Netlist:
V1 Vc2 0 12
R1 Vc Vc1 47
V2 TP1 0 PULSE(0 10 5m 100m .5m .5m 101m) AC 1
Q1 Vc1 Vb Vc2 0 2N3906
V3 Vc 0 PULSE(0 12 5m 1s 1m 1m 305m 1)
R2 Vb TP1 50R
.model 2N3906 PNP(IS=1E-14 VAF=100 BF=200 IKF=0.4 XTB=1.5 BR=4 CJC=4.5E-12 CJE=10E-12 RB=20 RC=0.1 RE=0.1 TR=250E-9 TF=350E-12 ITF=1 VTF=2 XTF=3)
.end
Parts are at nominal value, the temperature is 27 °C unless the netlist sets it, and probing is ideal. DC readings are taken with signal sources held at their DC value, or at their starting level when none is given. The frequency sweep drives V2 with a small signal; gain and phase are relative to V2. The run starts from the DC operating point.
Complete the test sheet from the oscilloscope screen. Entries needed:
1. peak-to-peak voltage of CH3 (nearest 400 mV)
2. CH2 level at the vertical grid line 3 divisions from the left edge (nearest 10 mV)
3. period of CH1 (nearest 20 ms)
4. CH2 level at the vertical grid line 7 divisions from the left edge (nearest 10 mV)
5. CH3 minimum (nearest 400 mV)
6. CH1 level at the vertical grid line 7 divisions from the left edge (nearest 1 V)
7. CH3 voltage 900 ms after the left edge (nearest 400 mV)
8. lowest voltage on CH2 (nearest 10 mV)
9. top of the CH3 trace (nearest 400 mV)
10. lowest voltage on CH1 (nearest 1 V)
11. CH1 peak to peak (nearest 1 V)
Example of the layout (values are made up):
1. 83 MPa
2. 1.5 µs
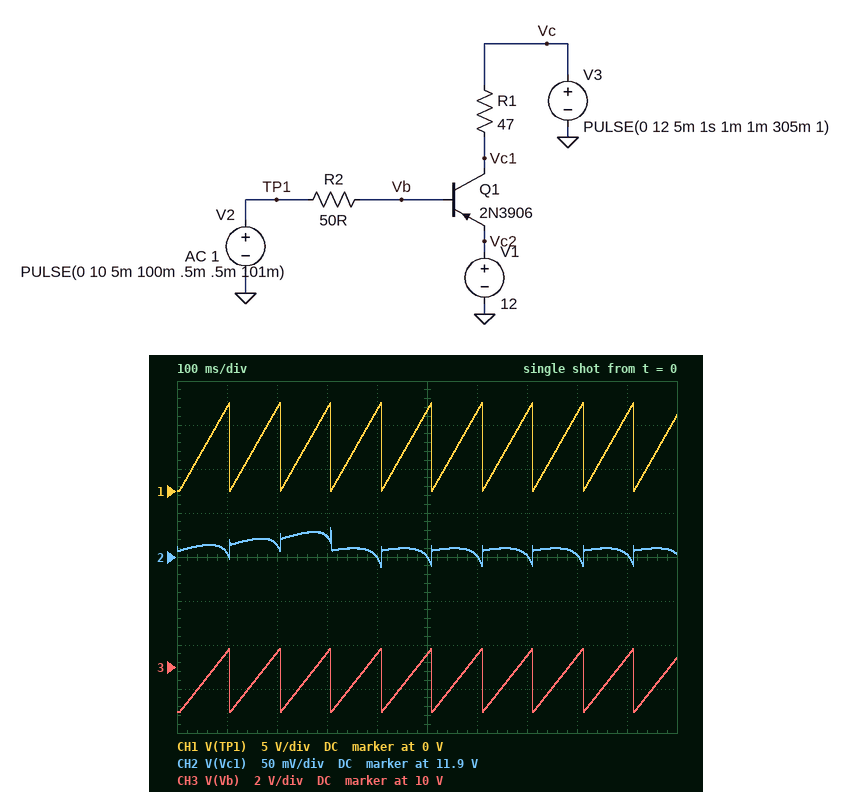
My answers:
1. 2.8 V
2. 11.92 V
3. 100 ms
4. 11.90 V
5. 8.0 V
6. 9 V
7. 10.4 V
8. 11.89 V
9. 10.8 V
10. 0 V
11. 10 V
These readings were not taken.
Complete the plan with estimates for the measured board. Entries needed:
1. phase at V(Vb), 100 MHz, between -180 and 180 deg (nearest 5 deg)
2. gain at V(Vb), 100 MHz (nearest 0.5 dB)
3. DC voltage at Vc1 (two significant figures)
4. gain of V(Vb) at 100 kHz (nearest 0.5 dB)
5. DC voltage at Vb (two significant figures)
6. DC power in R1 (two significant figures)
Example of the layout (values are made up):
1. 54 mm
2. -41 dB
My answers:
1. 0 deg
2. -11.0 dB
3. 12 V
4. -11.0 dB
5. 7.9 V
6. 3.0 W
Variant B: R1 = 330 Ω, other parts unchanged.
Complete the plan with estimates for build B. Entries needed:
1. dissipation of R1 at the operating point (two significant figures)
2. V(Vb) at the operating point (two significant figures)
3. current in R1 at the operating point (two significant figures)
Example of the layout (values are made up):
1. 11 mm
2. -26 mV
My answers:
1. 430 mW
2. 8.0 V
3. 36 mA
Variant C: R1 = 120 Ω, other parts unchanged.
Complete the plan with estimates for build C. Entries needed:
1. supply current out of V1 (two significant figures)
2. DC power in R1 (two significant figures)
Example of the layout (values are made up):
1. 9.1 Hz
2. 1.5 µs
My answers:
1. 260 mA
2. 1.2 W
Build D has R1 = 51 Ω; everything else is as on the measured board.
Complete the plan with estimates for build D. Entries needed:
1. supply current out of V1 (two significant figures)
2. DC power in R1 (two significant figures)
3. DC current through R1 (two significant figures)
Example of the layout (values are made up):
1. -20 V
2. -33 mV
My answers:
1. 390 mA
2. 2.8 W
3. 230 mA
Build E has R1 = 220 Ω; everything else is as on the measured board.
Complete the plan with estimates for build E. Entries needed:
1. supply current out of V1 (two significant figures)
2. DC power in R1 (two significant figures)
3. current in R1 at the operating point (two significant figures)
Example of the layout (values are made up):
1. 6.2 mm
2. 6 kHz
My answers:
1. 210 mA
2. 650 mW
3. 54 mA
